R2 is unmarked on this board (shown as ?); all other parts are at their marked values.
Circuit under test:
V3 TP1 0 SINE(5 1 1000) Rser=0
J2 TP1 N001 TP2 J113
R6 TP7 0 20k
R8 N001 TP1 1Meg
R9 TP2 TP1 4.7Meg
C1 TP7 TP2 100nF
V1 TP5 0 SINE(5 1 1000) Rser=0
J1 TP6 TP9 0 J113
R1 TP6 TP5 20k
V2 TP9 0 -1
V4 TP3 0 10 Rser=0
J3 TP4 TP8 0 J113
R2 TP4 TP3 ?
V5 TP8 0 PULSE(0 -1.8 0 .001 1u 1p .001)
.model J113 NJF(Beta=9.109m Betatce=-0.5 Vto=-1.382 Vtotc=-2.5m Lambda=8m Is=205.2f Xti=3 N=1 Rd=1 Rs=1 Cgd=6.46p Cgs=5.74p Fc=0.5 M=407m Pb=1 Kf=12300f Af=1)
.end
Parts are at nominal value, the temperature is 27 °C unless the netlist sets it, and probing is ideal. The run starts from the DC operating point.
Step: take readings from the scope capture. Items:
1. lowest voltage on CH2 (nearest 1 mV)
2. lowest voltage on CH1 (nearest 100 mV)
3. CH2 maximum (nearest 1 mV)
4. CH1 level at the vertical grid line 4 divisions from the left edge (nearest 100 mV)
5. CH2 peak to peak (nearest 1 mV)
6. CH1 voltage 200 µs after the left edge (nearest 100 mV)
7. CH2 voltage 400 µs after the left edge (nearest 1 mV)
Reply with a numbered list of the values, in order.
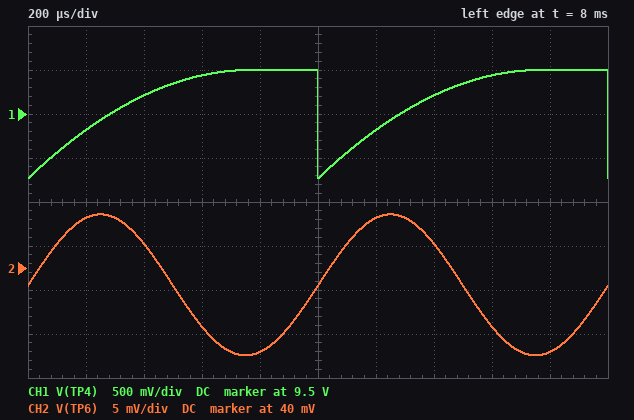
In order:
1. 30 mV
2. 8.8 V
3. 46 mV
4. 10.0 V
5. 16 mV
6. 9.3 V
7. 43 mV
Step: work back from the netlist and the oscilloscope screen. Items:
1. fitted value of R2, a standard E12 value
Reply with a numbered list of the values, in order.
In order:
1. 68 Ω
